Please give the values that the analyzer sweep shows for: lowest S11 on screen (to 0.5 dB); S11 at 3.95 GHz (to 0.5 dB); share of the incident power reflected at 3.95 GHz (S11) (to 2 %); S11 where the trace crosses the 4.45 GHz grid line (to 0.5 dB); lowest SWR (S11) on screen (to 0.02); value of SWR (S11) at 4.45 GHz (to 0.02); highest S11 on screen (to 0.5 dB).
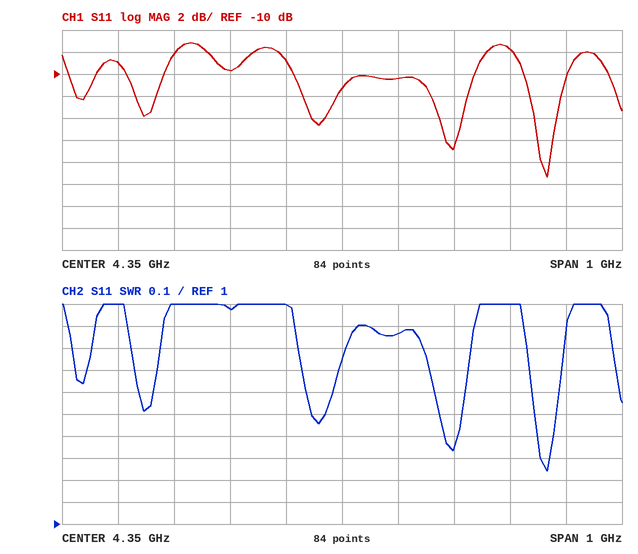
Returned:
-19.5 dB
-9.0 dB
12 %
-10.5 dB
1.24
1.86
-7.0 dB
